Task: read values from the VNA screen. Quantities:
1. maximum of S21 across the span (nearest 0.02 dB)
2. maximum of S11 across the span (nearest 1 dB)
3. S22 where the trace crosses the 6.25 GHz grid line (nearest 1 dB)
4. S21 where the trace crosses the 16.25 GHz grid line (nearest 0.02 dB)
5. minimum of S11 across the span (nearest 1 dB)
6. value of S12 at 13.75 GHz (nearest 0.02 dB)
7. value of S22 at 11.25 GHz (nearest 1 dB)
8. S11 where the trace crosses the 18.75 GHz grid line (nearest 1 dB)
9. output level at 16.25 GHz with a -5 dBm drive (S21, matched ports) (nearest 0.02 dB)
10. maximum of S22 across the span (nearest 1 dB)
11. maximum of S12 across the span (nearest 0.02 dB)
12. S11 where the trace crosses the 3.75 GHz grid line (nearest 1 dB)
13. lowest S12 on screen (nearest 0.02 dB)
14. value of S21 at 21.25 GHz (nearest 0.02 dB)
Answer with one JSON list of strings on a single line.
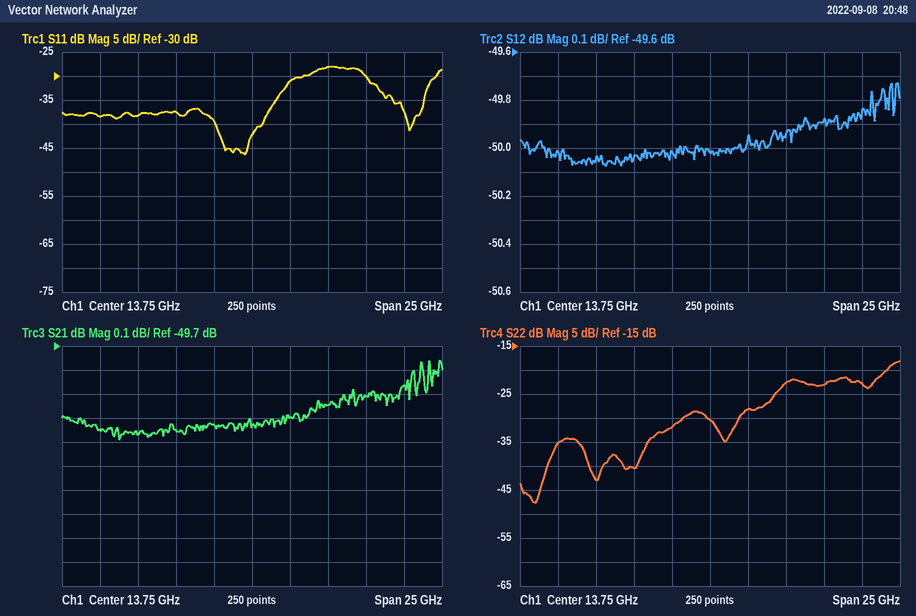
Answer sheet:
["-49.76 dB", "-28 dB", "-43 dB", "-50.00 dB", "-46 dB", "-50.02 dB", "-32 dB", "-28 dB", "-55.00 dBm", "-18 dB", "-49.72 dB", "-38 dB", "-50.08 dB", "-49.90 dB"]
